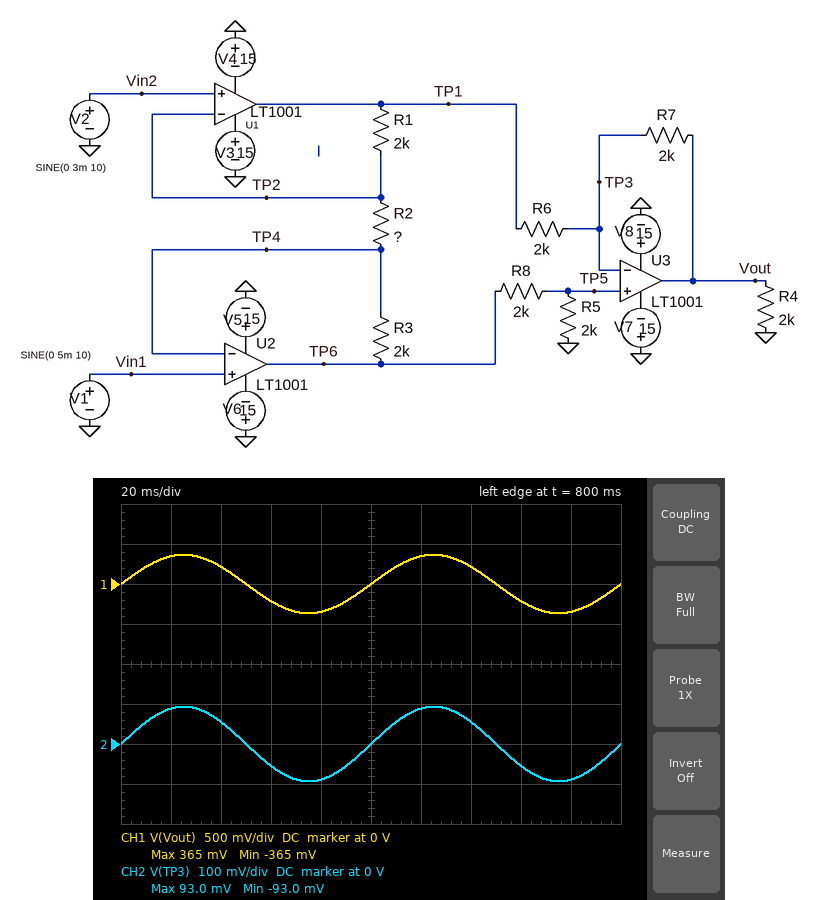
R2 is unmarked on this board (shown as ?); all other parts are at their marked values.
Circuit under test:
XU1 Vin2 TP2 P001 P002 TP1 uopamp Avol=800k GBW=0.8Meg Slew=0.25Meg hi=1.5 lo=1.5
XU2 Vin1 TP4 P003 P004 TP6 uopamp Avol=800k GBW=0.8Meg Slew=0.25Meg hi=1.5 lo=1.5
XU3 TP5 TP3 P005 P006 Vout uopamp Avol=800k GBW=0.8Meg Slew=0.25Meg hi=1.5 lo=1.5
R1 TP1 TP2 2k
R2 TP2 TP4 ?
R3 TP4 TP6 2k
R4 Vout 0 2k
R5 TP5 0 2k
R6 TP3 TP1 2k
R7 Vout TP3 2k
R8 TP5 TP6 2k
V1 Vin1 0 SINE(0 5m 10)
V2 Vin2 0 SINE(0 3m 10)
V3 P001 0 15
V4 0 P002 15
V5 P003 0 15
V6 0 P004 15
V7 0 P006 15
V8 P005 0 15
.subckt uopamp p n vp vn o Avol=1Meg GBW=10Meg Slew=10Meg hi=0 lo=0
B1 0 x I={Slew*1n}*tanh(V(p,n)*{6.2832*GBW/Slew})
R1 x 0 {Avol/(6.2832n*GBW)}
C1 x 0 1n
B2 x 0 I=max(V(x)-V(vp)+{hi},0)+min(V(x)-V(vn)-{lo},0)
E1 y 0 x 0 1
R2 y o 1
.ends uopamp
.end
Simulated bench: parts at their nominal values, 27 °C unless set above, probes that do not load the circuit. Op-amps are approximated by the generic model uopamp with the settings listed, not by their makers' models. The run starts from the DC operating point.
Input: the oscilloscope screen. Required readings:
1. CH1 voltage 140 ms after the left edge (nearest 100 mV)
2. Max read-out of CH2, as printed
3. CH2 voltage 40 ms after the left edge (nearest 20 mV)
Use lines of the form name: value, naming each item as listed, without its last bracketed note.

CH1 voltage 140 ms after the left edge: 200 mV
Max read-out of CH2, as printed: 93.0 mV
CH2 voltage 40 ms after the left edge: 60 mV
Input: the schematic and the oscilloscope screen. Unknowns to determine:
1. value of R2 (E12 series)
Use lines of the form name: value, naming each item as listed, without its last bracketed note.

value of R2: 22 Ω
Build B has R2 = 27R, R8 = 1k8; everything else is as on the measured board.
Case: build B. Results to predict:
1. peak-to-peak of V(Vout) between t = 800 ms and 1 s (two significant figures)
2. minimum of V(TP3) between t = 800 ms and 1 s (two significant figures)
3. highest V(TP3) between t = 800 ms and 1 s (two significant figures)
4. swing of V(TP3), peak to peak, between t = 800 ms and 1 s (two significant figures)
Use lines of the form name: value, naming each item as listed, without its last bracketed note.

peak-to-peak of V(Vout) between t = 800 ms and 1 s: 610 mV
minimum of V(TP3) between t = 800 ms and 1 s: -81 mV
highest V(TP3) between t = 800 ms and 1 s: 81 mV
swing of V(TP3), peak to peak, between t = 800 ms and 1 s: 160 mV
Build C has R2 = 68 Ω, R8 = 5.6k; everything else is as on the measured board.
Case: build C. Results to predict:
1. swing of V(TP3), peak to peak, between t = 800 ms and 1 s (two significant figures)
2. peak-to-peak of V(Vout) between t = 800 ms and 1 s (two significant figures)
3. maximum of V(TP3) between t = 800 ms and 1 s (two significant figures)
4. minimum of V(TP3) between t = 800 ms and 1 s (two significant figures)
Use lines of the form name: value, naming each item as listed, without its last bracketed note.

swing of V(TP3), peak to peak, between t = 800 ms and 1 s: 34 mV
peak-to-peak of V(Vout) between t = 800 ms and 1 s: 180 mV
maximum of V(TP3) between t = 800 ms and 1 s: 17 mV
minimum of V(TP3) between t = 800 ms and 1 s: -17 mV
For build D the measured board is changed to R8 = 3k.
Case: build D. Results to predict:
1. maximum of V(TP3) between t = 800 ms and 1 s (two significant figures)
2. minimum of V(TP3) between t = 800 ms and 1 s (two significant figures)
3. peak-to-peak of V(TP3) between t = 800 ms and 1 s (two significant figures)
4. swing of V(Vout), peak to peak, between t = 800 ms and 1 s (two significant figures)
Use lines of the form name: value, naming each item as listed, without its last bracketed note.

maximum of V(TP3) between t = 800 ms and 1 s: 75 mV
minimum of V(TP3) between t = 800 ms and 1 s: -75 mV
peak-to-peak of V(TP3) between t = 800 ms and 1 s: 150 mV
swing of V(Vout), peak to peak, between t = 800 ms and 1 s: 660 mV
